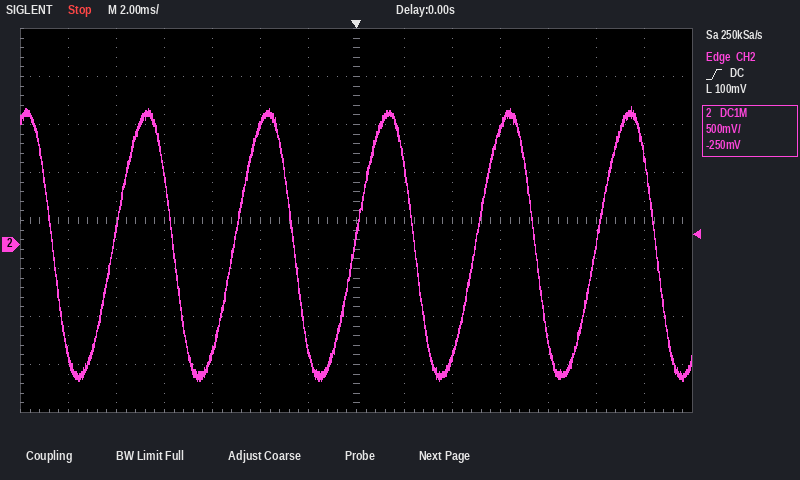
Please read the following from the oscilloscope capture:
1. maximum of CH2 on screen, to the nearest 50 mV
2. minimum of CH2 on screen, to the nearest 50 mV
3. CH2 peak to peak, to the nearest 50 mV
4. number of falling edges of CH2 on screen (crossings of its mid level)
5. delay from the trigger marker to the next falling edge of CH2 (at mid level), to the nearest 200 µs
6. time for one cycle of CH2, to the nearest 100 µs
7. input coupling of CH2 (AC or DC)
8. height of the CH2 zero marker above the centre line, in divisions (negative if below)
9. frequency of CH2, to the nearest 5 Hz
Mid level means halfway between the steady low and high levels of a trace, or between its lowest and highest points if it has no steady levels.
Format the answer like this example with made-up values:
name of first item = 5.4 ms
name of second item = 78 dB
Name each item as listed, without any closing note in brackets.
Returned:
maximum of CH2 on screen, to the nearest 50 mV = 1.45 V
minimum of CH2 on screen, to the nearest 50 mV = -1.40 V
CH2 peak to peak, to the nearest 50 mV = 2.85 V
number of falling edges of CH2 on screen = 6
delay from the trigger marker to the next falling edge of CH2 (at mid level), to the nearest 200 µs = 2.4 ms
time for one cycle of CH2, to the nearest 100 µs = 5.0 ms
input coupling of CH2 = DC
height of the CH2 zero marker above the centre line, in divisions = -0.5 div
frequency of CH2, to the nearest 5 Hz = 200 Hz
